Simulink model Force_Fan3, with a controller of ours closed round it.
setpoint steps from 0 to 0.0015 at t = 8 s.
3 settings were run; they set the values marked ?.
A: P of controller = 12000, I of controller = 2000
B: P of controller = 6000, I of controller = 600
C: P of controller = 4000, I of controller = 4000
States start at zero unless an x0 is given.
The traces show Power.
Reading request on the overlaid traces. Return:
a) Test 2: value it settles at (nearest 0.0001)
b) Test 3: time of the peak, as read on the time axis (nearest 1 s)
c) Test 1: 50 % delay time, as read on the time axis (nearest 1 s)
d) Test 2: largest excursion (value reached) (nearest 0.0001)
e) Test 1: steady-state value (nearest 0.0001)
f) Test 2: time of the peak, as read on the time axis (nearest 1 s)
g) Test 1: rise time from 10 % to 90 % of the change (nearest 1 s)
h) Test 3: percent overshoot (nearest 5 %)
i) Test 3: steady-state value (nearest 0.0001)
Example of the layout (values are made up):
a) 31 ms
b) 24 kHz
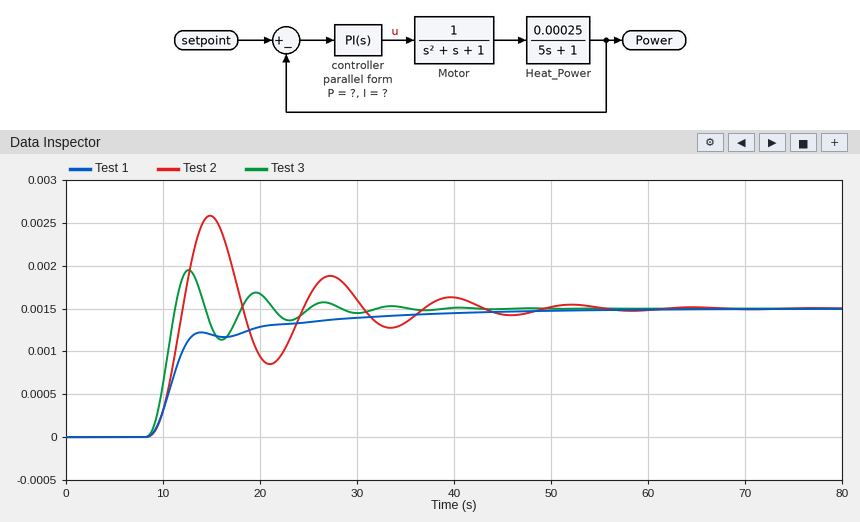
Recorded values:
a) 0.0015
b) 13 s
c) 11 s
d) 0.0026
e) 0.0015
f) 15 s
g) 16 s
h) 30 %
i) 0.0015
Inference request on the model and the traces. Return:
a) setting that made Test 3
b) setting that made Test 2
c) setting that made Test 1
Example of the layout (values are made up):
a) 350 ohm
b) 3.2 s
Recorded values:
a) A
b) C
c) B
